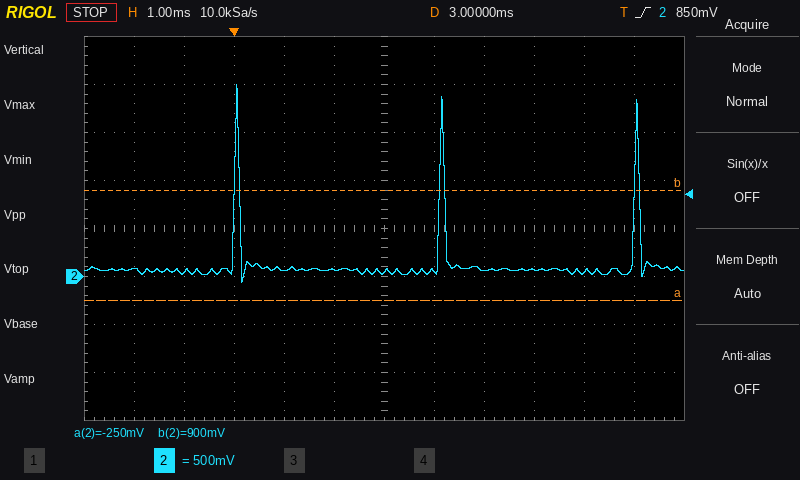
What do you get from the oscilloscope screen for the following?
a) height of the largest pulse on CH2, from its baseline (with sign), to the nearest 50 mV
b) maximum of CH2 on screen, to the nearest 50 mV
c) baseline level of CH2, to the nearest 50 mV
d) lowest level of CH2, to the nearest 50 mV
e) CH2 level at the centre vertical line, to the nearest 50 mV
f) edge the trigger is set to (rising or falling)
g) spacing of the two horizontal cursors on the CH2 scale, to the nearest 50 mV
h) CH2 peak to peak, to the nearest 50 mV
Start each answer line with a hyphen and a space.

- +1.95 V
- 2.00 V
- 50 mV
- -50 mV
- 50 mV
- rising
- 1.15 V
- 2.05 V
